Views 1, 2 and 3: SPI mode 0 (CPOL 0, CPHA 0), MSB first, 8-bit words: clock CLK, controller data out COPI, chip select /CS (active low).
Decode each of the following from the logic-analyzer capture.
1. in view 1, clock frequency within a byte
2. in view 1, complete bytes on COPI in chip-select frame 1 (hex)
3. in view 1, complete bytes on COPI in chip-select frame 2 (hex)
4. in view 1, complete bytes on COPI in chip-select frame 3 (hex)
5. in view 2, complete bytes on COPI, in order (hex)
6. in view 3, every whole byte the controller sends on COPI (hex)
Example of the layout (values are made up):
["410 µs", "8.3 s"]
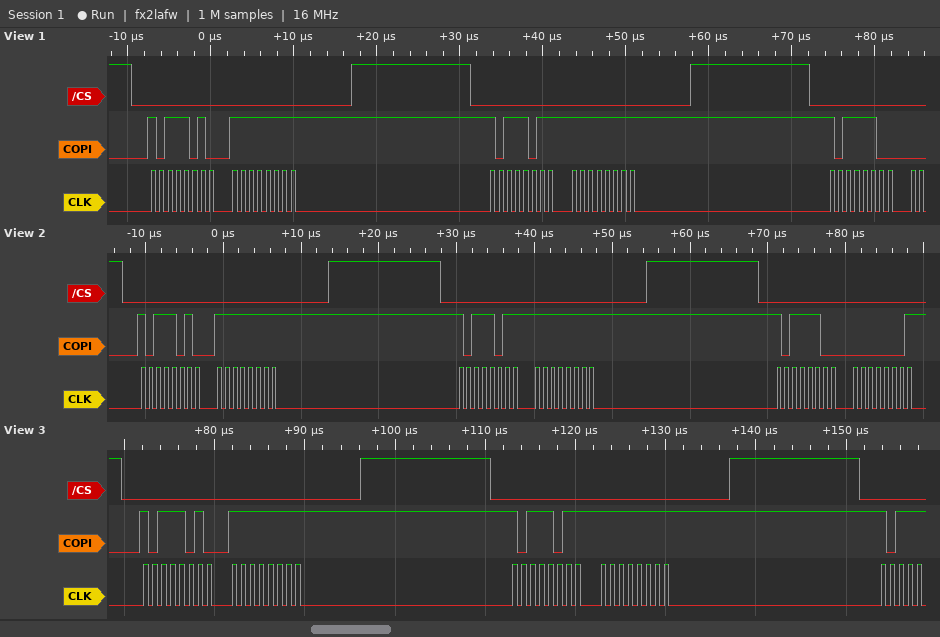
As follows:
["1 MHz", "BA FF", "BB FF", "BC", "0xBA 0xFF 0xBB 0xFF 0xBC 0x01", "BA FF BB FF"]
